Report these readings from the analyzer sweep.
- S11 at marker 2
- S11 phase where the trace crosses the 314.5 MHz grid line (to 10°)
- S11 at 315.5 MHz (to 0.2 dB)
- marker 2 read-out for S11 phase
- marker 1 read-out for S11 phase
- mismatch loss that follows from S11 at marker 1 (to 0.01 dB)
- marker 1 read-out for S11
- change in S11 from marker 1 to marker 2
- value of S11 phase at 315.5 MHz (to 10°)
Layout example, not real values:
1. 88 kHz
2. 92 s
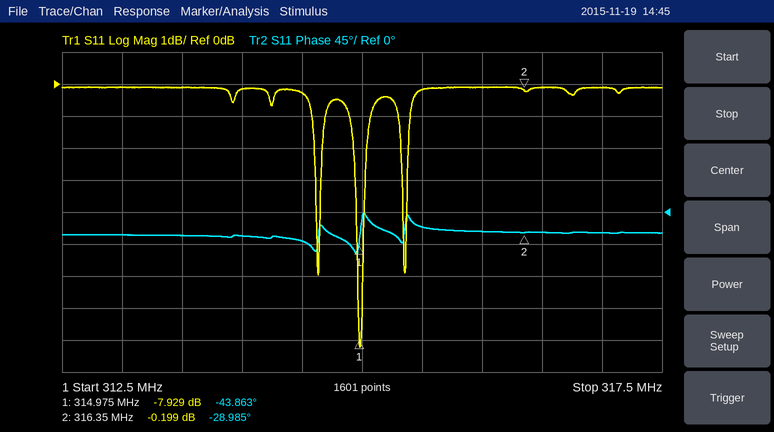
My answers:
1. -0.199 dB
2. -40°
3. -0.2 dB
4. -28.985°
5. -43.863°
6. 0.76 dB
7. -7.929 dB
8. 7.730 dB
9. -20°
